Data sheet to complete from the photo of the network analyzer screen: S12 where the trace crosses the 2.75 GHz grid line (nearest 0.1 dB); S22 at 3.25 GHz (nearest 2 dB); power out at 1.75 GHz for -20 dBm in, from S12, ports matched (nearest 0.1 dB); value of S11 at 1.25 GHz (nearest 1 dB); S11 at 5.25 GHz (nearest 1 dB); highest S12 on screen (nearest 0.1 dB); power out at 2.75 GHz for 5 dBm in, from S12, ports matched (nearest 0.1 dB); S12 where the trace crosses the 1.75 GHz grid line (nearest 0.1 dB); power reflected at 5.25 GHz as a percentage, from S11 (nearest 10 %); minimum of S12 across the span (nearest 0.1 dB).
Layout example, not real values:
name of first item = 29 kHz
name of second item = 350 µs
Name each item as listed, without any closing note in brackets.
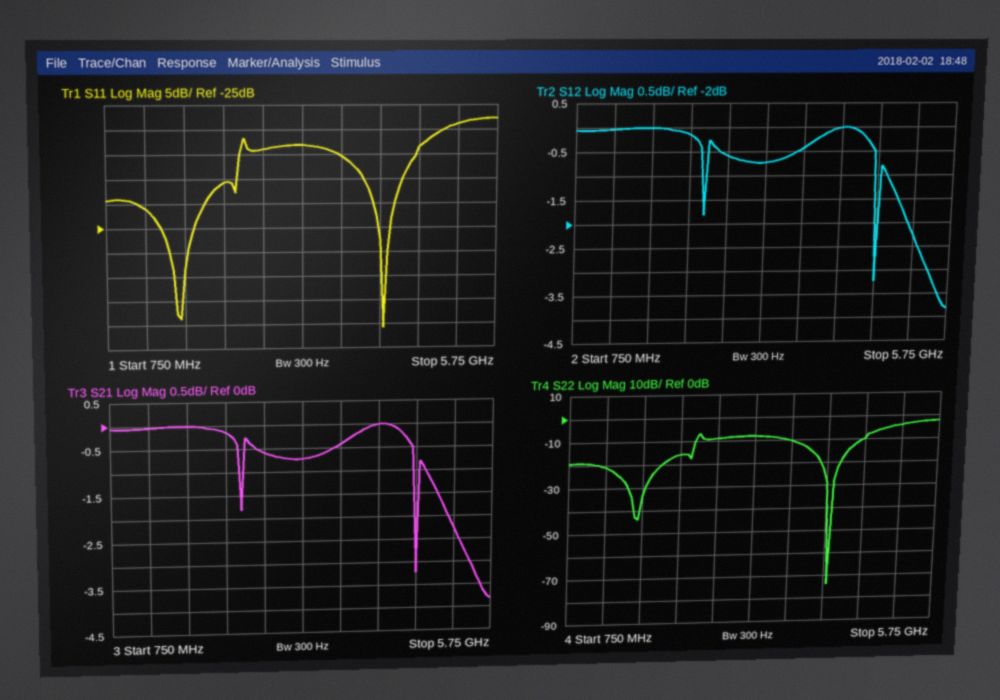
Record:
S12 where the trace crosses the 2.75 GHz grid line = -0.6 dB
S22 at 3.25 GHz = -8 dB
power out at 1.75 GHz for -20 dBm in, from S12, ports matched = -20.0 dBm
value of S11 at 1.25 GHz = -21 dB
S11 at 5.25 GHz = -4 dB
highest S12 on screen = 0.0 dB
power out at 2.75 GHz for 5 dBm in, from S12, ports matched = 4.4 dBm
S12 where the trace crosses the 1.75 GHz grid line = 0.0 dB
power reflected at 5.25 GHz as a percentage, from S11 = 40 %
minimum of S12 across the span = -3.8 dB
